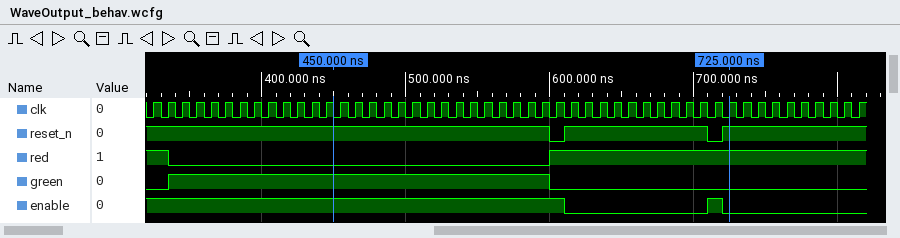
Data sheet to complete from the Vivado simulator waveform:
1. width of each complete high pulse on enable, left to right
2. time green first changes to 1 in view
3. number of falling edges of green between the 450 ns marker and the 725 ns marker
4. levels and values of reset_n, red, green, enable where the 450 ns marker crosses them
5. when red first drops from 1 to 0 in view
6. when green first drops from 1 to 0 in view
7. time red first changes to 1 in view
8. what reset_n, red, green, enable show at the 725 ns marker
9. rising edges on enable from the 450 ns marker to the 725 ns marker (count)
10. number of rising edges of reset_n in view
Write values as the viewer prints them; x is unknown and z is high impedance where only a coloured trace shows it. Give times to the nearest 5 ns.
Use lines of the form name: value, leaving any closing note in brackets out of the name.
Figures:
width of each complete high pulse on enable, left to right: 10 ns
time green first changes to 1 in view: 335 ns
number of falling edges of green between the 450 ns marker and the 725 ns marker: 1
levels and values of reset_n, red, green, enable where the 450 ns marker crosses them: reset_n=1, red=0, green=1, enable=1
when red first drops from 1 to 0 in view: 335 ns
when green first drops from 1 to 0 in view: 600 ns
time red first changes to 1 in view: 600 ns
what reset_n, red, green, enable show at the 725 ns marker: reset_n=1, red=1, green=0, enable=0
rising edges on enable from the 450 ns marker to the 725 ns marker: 1
number of rising edges of reset_n in view: 2
